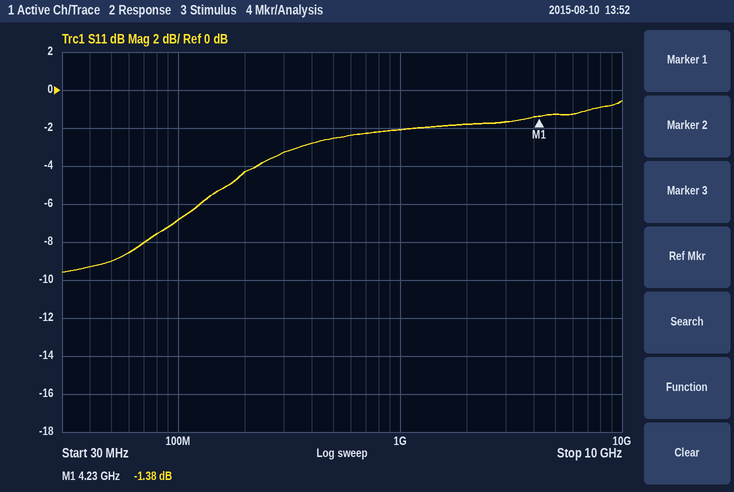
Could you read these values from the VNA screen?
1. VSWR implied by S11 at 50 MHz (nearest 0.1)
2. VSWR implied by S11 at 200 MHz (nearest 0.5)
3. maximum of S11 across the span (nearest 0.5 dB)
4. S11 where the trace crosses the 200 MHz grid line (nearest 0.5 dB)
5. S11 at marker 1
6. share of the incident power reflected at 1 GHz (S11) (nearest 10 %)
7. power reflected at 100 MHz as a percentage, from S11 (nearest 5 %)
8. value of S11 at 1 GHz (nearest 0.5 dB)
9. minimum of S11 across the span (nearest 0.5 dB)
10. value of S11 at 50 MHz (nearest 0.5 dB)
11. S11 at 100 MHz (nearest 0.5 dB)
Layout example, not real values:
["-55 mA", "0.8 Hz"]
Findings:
["2.1", "4.0", "-0.5 dB", "-4.5 dB", "-1.38 dB", "60 %", "20 %", "-2.0 dB", "-9.5 dB", "-9.0 dB", "-7.0 dB"]
